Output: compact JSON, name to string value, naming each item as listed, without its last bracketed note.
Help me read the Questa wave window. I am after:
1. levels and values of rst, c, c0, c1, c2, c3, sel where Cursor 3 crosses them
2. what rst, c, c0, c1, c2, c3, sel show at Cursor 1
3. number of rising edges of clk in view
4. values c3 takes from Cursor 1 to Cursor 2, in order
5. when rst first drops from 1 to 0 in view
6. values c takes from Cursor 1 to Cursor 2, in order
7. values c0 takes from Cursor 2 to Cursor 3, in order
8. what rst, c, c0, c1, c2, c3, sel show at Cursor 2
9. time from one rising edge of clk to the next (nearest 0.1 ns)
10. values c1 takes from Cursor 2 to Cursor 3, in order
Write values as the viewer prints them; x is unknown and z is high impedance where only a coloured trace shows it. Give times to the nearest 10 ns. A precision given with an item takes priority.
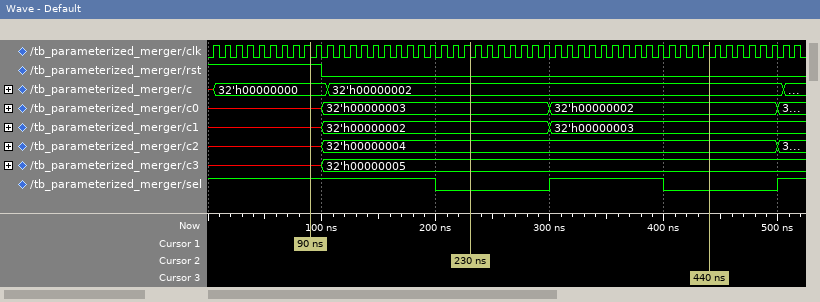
{"levels and values of rst, c, c0, c1, c2, c3, sel where Cursor 3 crosses them": "rst=0, c=32'h00000002, c0=32'h00000002, c1=32'h00000003, c2=32'h00000004, c3=32'h00000005, sel=0", "what rst, c, c0, c1, c2, c3, sel show at Cursor 1": "rst=1, c=32'h00000000, c0=x, c1=x, c2=x, c3=x, sel=1", "number of rising edges of clk in view": "52", "values c3 takes from Cursor 1 to Cursor 2, in order": "x, 32'h00000005", "when rst first drops from 1 to 0 in view": "100 ns", "values c takes from Cursor 1 to Cursor 2, in order": "32'h00000000, 32'h00000002", "values c0 takes from Cursor 2 to Cursor 3, in order": "32'h00000003, 32'h00000002", "what rst, c, c0, c1, c2, c3, sel show at Cursor 2": "rst=0, c=32'h00000002, c0=32'h00000003, c1=32'h00000002, c2=32'h00000004, c3=32'h00000005, sel=0", "time from one rising edge of clk to the next": "10 ns", "values c1 takes from Cursor 2 to Cursor 3, in order": "32'h00000002, 32'h00000003"}
